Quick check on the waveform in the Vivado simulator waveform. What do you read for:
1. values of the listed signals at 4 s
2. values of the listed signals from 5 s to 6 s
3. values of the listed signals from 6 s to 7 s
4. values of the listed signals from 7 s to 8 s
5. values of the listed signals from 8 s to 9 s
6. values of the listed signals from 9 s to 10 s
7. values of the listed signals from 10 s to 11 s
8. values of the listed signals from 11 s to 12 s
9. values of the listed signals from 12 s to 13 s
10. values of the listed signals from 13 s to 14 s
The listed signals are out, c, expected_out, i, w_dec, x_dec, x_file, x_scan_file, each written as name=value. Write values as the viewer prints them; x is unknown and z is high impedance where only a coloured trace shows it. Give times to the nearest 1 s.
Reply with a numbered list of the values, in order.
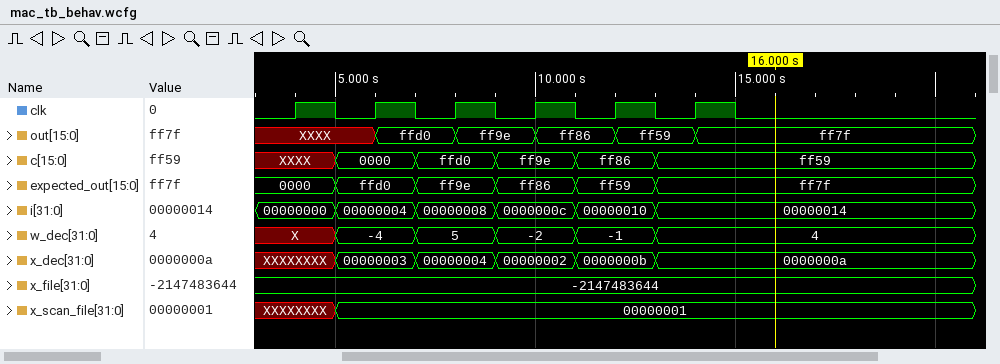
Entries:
1. out=XXXX, c=XXXX, expected_out=0000, i=00000000, w_dec=X, x_dec=XXXXXXXX, x_file=-2147483644, x_scan_file=XXXXXXXX
2. out=XXXX, c=0000, expected_out=ffd0, i=00000004, w_dec=-4, x_dec=00000003, x_file=-2147483644, x_scan_file=00000001
3. out=ffd0, c=0000, expected_out=ffd0, i=00000004, w_dec=-4, x_dec=00000003, x_file=-2147483644, x_scan_file=00000001
4. out=ffd0, c=ffd0, expected_out=ff9e, i=00000008, w_dec=5, x_dec=00000004, x_file=-2147483644, x_scan_file=00000001
5. out=ff9e, c=ffd0, expected_out=ff9e, i=00000008, w_dec=5, x_dec=00000004, x_file=-2147483644, x_scan_file=00000001
6. out=ff9e, c=ff9e, expected_out=ff86, i=0000000c, w_dec=-2, x_dec=00000002, x_file=-2147483644, x_scan_file=00000001
7. out=ff86, c=ff9e, expected_out=ff86, i=0000000c, w_dec=-2, x_dec=00000002, x_file=-2147483644, x_scan_file=00000001
8. out=ff86, c=ff86, expected_out=ff59, i=00000010, w_dec=-1, x_dec=0000000b, x_file=-2147483644, x_scan_file=00000001
9. out=ff59, c=ff86, expected_out=ff59, i=00000010, w_dec=-1, x_dec=0000000b, x_file=-2147483644, x_scan_file=00000001
10. out=ff59, c=ff59, expected_out=ff7f, i=00000014, w_dec=4, x_dec=0000000a, x_file=-2147483644, x_scan_file=00000001
